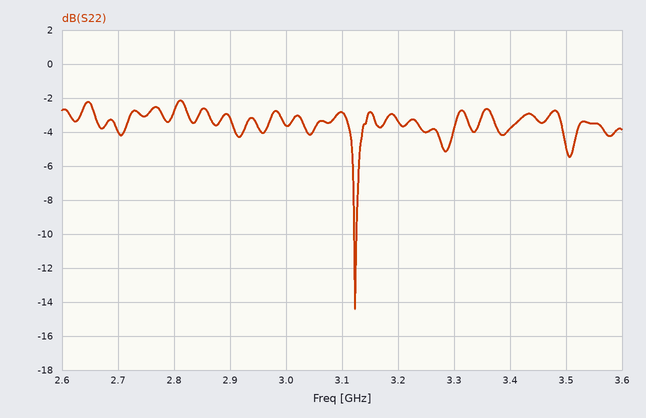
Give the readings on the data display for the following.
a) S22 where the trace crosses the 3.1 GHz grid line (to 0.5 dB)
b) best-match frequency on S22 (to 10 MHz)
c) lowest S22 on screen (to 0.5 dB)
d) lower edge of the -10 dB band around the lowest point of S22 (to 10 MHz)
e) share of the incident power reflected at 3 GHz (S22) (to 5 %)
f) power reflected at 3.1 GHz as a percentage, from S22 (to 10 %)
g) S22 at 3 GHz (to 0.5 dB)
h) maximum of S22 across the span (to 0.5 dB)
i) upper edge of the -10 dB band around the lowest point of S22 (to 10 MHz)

-3.0 dB
3.12 GHz
-14.5 dB
3.12 GHz
45 %
50 %
-3.5 dB
-2.0 dB
3.13 GHz
